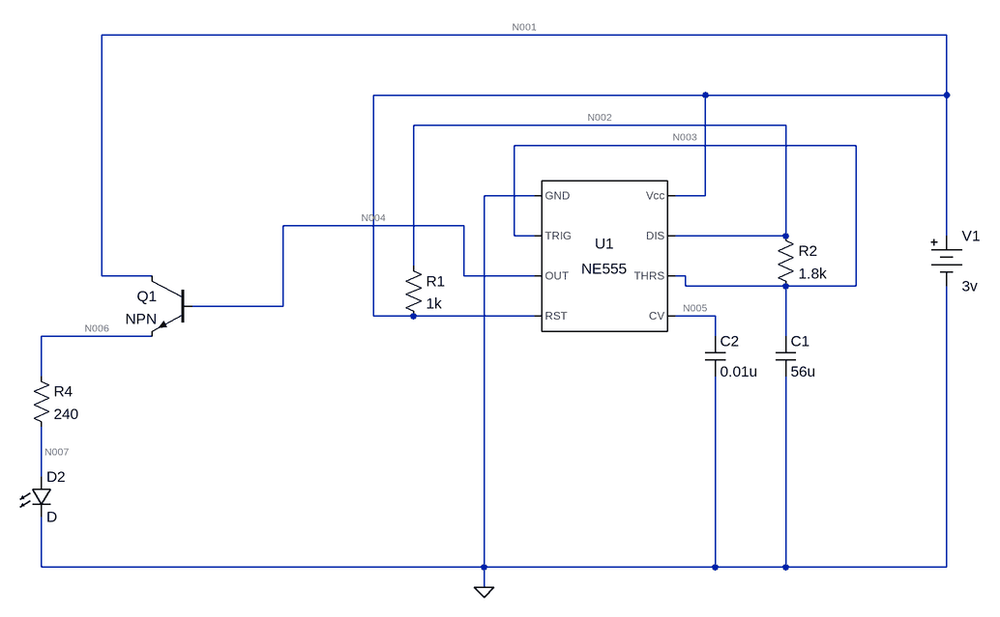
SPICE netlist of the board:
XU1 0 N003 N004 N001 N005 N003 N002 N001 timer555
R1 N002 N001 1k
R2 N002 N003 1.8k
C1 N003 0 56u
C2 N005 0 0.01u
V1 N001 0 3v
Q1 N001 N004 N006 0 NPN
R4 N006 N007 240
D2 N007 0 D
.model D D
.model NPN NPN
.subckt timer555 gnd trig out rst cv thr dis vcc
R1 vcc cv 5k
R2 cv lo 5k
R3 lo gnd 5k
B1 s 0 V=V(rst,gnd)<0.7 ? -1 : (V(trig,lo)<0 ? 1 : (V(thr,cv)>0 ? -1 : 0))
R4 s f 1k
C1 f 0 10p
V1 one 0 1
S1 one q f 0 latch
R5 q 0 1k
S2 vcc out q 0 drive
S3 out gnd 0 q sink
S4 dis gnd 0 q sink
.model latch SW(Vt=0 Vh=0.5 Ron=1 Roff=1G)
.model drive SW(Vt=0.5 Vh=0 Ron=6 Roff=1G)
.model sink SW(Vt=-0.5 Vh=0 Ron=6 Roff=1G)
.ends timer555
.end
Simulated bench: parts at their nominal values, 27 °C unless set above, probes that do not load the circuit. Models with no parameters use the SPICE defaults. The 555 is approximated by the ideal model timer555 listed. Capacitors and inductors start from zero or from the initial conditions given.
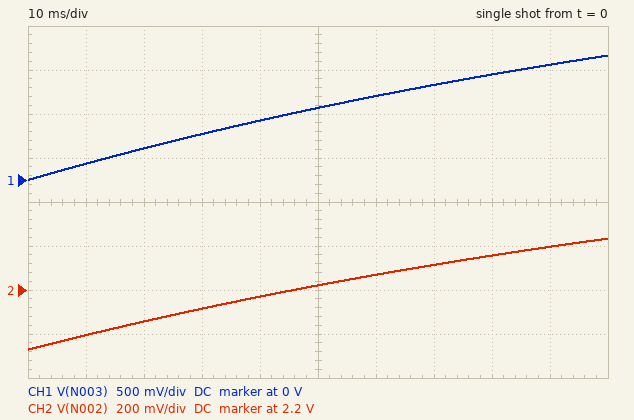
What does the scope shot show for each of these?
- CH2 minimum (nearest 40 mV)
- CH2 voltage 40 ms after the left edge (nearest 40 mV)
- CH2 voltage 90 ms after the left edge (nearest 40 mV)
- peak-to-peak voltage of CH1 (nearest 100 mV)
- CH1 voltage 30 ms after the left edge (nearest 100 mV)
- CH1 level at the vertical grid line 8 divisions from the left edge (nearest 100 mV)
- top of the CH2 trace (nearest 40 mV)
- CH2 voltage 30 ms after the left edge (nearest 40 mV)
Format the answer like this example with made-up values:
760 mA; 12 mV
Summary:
1.92 V; 2.16 V; 2.40 V; 1.4 V; 500 mV; 1.2 V; 2.44 V; 2.12 V
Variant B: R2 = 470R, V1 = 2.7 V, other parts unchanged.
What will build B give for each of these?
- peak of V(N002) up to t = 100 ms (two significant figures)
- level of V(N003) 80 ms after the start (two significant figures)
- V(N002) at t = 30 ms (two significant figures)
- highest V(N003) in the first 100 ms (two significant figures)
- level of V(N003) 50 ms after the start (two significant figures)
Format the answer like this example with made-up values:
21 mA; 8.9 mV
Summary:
2.1 V; 1.7 V; 1.4 V; 1.8 V; 1.2 V
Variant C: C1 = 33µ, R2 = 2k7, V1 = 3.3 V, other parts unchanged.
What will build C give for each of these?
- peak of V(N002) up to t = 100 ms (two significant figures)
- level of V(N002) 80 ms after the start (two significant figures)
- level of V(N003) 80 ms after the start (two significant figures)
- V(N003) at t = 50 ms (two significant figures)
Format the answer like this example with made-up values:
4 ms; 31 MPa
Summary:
2.9 V; 2.8 V; 1.6 V; 1.1 V
